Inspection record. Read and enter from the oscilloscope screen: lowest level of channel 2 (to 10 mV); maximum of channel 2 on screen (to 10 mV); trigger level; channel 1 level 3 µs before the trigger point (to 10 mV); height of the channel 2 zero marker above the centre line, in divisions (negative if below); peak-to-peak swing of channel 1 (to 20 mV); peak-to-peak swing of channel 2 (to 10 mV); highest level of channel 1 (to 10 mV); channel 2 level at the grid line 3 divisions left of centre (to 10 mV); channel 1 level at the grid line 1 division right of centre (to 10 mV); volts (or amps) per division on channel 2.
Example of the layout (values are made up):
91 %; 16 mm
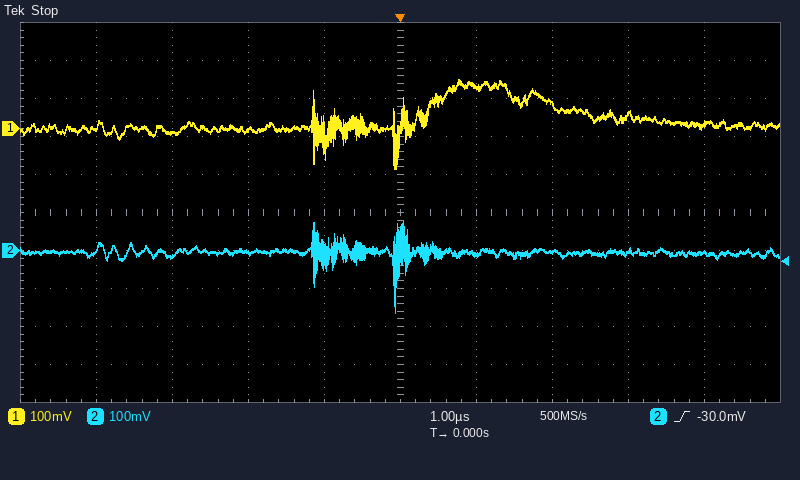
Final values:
-160 mV; 80 mV; -30.0 mV; -10 mV; -1.0 div; 240 mV; 240 mV; 130 mV; -10 mV; 110 mV; 100 mV
